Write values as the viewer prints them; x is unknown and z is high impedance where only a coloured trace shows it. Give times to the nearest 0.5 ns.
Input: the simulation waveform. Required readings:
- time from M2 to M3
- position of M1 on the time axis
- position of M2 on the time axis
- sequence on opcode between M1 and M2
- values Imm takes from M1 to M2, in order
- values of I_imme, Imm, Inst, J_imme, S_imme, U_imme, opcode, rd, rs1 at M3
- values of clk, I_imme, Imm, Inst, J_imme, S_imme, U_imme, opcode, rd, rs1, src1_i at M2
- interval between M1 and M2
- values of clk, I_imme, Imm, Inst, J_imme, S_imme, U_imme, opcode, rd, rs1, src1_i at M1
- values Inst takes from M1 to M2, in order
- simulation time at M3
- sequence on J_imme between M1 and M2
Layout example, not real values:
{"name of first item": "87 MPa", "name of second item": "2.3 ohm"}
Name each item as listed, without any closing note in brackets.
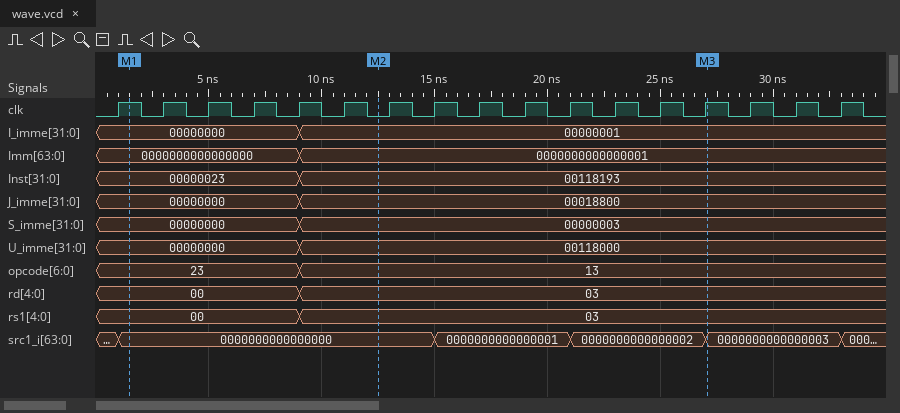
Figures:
{"time from M2 to M3": "14.5 ns", "position of M1 on the time axis": "1.5 ns", "position of M2 on the time axis": "12.5 ns", "sequence on opcode between M1 and M2": "23, 13", "values Imm takes from M1 to M2, in order": "0000000000000000, 0000000000000001", "values of I_imme, Imm, Inst, J_imme, S_imme, U_imme, opcode, rd, rs1 at M3": "I_imme=00000001, Imm=0000000000000001, Inst=00118193, J_imme=00018800, S_imme=00000003, U_imme=00118000, opcode=13, rd=03, rs1=03", "values of clk, I_imme, Imm, Inst, J_imme, S_imme, U_imme, opcode, rd, rs1, src1_i at M2": "clk=0, I_imme=00000001, Imm=0000000000000001, Inst=00118193, J_imme=00018800, S_imme=00000003, U_imme=00118000, opcode=13, rd=03, rs1=03, src1_i=0000000000000000", "interval between M1 and M2": "11 ns", "values of clk, I_imme, Imm, Inst, J_imme, S_imme, U_imme, opcode, rd, rs1, src1_i at M1": "clk=1, I_imme=00000000, Imm=0000000000000000, Inst=00000023, J_imme=00000000, S_imme=00000000, U_imme=00000000, opcode=23, rd=00, rs1=00, src1_i=0000000000000000", "values Inst takes from M1 to M2, in order": "00000023, 00118193", "simulation time at M3": "27 ns", "sequence on J_imme between M1 and M2": "00000000, 00018800"}
